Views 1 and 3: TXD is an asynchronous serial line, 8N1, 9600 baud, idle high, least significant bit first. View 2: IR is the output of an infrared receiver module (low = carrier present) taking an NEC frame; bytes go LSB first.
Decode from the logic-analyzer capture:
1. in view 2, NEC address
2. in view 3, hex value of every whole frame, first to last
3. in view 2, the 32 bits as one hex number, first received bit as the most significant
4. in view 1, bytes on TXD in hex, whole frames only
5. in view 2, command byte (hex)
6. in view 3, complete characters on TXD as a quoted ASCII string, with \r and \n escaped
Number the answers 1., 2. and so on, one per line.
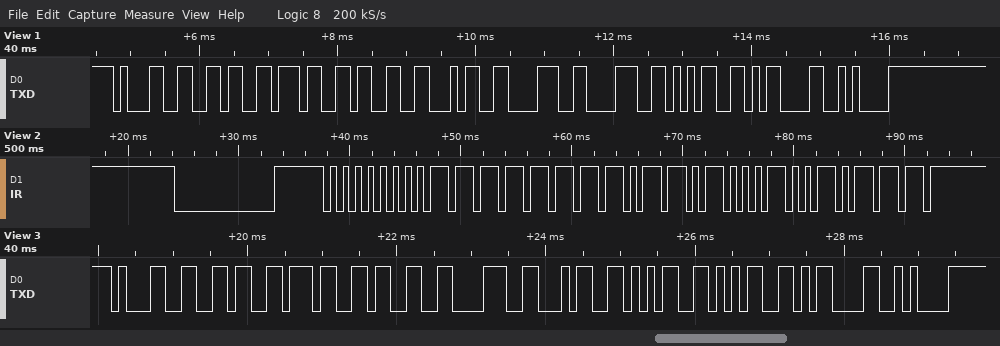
1. 0x00
2. 31 36 37 33 38 34 35 35 0D 0A
3. 0x00FF6897
4. 31 36 37 33 34 38 38 35 0D 0A
5. 0x16
6. "16738455\r\n"
